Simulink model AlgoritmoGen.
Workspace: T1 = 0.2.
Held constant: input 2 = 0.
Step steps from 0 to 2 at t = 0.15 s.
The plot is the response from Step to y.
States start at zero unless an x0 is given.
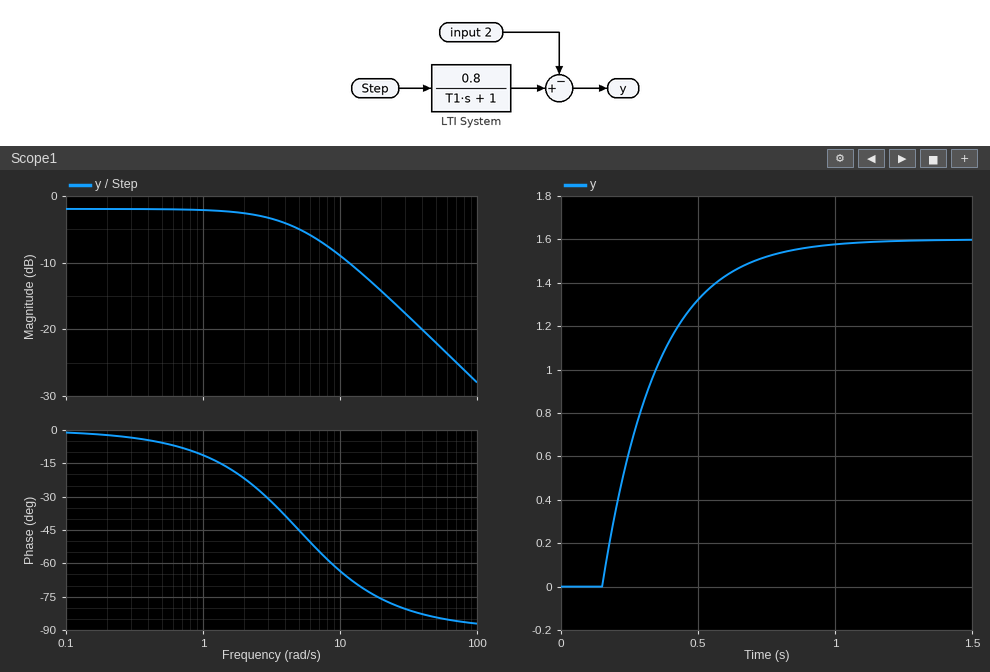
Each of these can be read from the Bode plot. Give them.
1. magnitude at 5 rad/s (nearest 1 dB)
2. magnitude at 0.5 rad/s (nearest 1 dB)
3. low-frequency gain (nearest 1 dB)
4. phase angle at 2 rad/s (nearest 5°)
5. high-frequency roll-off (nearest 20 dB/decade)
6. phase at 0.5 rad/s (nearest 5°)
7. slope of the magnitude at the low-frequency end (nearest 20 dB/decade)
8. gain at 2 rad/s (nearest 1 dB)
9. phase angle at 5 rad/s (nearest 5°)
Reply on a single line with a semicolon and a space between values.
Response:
-5 dB; -2 dB; -2 dB; -20°; -20 dB/decade; -5°; 0 dB/decade; -3 dB; -45°
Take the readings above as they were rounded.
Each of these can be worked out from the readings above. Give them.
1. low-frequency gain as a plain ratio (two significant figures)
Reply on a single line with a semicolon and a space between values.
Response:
0.79
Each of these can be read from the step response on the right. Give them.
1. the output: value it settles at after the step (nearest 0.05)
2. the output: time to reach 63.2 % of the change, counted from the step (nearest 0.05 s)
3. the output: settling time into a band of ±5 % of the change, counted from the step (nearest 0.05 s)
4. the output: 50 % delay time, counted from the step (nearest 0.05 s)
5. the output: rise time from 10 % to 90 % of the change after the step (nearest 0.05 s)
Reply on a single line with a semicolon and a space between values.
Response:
1.60; 0.20 s; 0.60 s; 0.15 s; 0.45 s
